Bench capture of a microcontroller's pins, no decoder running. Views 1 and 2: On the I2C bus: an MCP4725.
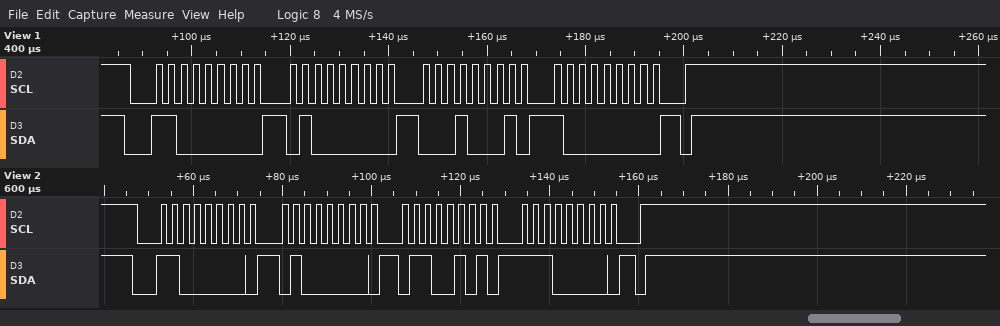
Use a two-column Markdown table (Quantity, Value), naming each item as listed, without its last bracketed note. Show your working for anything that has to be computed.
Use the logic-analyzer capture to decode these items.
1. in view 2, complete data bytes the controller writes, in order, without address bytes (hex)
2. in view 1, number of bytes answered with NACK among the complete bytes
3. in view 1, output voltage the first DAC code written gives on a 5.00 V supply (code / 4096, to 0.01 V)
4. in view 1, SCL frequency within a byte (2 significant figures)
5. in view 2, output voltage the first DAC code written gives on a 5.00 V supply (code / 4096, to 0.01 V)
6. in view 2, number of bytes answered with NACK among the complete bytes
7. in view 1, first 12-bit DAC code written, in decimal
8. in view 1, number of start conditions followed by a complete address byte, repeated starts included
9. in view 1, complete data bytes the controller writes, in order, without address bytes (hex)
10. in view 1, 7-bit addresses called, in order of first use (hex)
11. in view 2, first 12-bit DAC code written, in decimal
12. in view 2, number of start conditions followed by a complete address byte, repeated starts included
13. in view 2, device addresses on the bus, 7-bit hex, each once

| Quantity | Value |
|---|---|
| in view 2, complete data bytes the controller writes, in order, without address bytes | 40 65 E0 |
| in view 1, number of bytes answered with NACK among the complete bytes | 0 |
| in view 1, output voltage the first DAC code written gives on a 5.00 V supply | 280 / 4096 x 5.00 V = 0.34 V |
| in view 1, SCL frequency within a byte | 400 kHz |
| in view 2, output voltage the first DAC code written gives on a 5.00 V supply | 1630 / 4096 x 5.00 V = 1.99 V |
| in view 2, number of bytes answered with NACK among the complete bytes | 0 |
| in view 1, first 12-bit DAC code written, in decimal | 280 |
| in view 1, number of start conditions followed by a complete address byte, repeated starts included | 1 |
| in view 1, complete data bytes the controller writes, in order, without address bytes | 40 11 80 |
| in view 1, 7-bit addresses called, in order of first use | 0x60 |
| in view 2, first 12-bit DAC code written, in decimal | 1630 |
| in view 2, number of start conditions followed by a complete address byte, repeated starts included | 1 |
| in view 2, device addresses on the bus, 7-bit hex, each once | 0x60 |
